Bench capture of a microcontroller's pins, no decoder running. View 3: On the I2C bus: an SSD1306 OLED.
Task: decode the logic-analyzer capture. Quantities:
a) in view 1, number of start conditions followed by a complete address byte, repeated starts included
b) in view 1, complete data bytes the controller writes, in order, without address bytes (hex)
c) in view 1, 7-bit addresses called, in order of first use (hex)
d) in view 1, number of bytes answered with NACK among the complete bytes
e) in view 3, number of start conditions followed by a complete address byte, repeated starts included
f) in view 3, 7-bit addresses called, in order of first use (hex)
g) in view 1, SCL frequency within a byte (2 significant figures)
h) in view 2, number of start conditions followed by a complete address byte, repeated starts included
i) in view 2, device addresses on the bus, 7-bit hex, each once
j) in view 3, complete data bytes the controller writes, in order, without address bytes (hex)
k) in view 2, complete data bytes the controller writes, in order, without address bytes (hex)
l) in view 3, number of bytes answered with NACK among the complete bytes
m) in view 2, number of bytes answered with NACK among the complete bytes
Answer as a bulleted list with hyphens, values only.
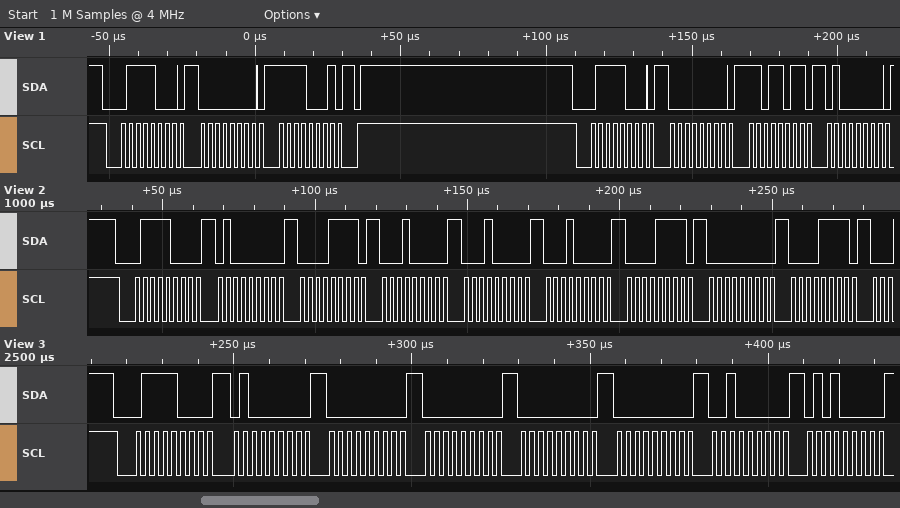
- 2
- 00 F1 00 DB 40
- 0x3C
- 0
- 1
- 0x3C
- 400 kHz
- 1
- 0x3C
- 40 00 00 00 00 20 50
- 40 0F 10 10 10 0F 00 0F
- 0
- 0
